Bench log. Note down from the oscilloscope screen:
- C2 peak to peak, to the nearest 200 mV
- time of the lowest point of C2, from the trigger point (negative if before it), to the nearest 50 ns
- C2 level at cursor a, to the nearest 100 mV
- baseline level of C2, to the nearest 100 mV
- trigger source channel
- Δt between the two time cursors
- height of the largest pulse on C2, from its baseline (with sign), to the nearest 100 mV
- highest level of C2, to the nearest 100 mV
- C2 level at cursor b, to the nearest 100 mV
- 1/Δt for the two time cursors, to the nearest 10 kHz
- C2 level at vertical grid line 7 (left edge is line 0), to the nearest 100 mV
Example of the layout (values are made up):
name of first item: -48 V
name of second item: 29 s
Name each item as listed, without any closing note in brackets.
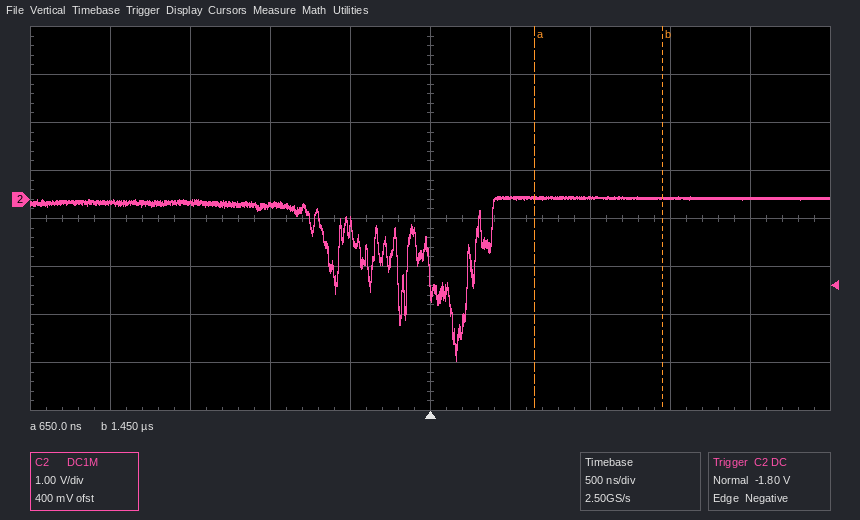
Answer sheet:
C2 peak to peak, to the nearest 200 mV: 3.4 V
time of the lowest point of C2, from the trigger point (negative if before it), to the nearest 50 ns: +150 ns
C2 level at cursor a, to the nearest 100 mV: 0.0 V
baseline level of C2, to the nearest 100 mV: 0.0 V
trigger source channel: C2
Δt between the two time cursors: 800 ns
height of the largest pulse on C2, from its baseline (with sign), to the nearest 100 mV: -3.4 V
highest level of C2, to the nearest 100 mV: 100 mV
C2 level at cursor b, to the nearest 100 mV: 0.0 V
1/Δt for the two time cursors, to the nearest 10 kHz: 1.25 MHz
C2 level at vertical grid line 7 (left edge is line 0), to the nearest 100 mV: 0.0 V
